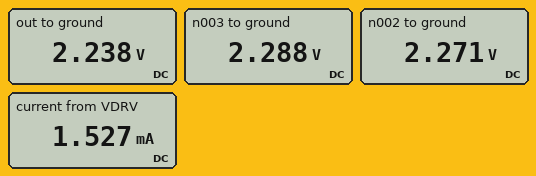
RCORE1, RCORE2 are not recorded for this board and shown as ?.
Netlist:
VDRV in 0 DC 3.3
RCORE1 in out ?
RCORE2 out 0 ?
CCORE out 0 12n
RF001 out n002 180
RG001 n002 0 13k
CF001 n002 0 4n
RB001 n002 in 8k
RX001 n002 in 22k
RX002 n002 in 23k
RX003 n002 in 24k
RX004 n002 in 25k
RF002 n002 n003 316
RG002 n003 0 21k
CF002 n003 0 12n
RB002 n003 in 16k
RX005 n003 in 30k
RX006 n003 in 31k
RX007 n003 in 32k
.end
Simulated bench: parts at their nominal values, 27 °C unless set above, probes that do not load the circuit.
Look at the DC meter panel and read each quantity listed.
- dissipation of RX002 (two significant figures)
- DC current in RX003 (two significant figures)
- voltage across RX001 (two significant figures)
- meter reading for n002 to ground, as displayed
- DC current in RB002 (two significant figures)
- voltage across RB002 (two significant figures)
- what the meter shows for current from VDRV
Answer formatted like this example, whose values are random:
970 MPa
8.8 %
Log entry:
46 µW
43 µA
1.0 V
2.271 V
63 µA
1.0 V
1.527 mA
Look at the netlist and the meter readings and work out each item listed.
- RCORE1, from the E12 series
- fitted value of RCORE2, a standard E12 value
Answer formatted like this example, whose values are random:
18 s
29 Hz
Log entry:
1 kΩ
1.8 kΩ
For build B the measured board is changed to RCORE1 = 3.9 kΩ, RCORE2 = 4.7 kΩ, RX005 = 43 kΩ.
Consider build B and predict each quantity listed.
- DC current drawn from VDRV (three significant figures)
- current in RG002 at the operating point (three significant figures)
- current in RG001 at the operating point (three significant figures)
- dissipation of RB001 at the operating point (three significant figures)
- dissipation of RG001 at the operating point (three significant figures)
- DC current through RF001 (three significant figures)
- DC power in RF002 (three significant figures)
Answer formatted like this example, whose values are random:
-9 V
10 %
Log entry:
749 µA
107 µA
172 µA
140 µW
386 µW
189 µA
740 nW
